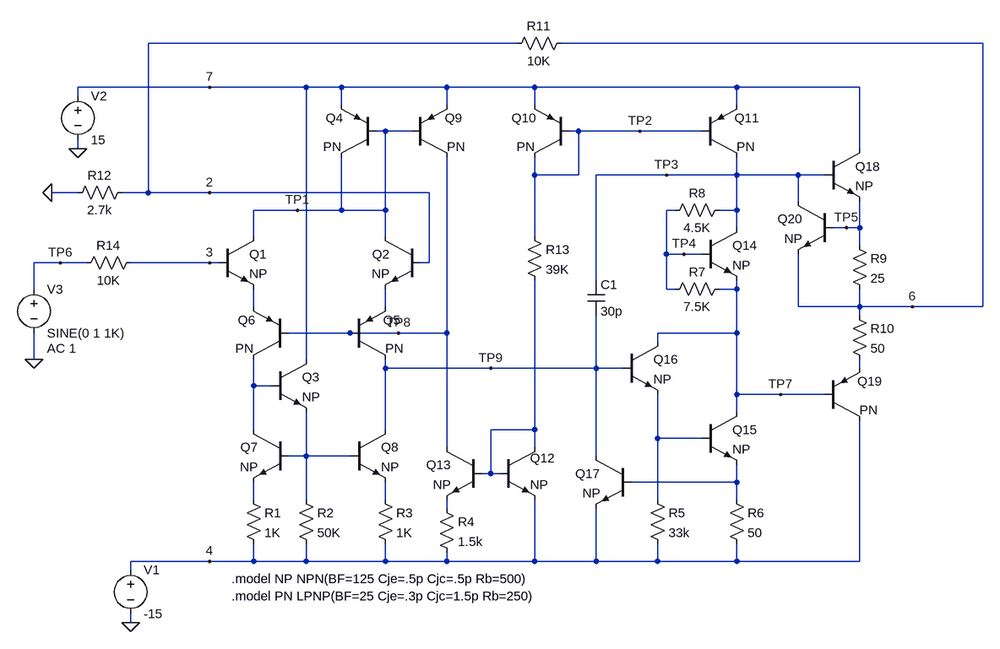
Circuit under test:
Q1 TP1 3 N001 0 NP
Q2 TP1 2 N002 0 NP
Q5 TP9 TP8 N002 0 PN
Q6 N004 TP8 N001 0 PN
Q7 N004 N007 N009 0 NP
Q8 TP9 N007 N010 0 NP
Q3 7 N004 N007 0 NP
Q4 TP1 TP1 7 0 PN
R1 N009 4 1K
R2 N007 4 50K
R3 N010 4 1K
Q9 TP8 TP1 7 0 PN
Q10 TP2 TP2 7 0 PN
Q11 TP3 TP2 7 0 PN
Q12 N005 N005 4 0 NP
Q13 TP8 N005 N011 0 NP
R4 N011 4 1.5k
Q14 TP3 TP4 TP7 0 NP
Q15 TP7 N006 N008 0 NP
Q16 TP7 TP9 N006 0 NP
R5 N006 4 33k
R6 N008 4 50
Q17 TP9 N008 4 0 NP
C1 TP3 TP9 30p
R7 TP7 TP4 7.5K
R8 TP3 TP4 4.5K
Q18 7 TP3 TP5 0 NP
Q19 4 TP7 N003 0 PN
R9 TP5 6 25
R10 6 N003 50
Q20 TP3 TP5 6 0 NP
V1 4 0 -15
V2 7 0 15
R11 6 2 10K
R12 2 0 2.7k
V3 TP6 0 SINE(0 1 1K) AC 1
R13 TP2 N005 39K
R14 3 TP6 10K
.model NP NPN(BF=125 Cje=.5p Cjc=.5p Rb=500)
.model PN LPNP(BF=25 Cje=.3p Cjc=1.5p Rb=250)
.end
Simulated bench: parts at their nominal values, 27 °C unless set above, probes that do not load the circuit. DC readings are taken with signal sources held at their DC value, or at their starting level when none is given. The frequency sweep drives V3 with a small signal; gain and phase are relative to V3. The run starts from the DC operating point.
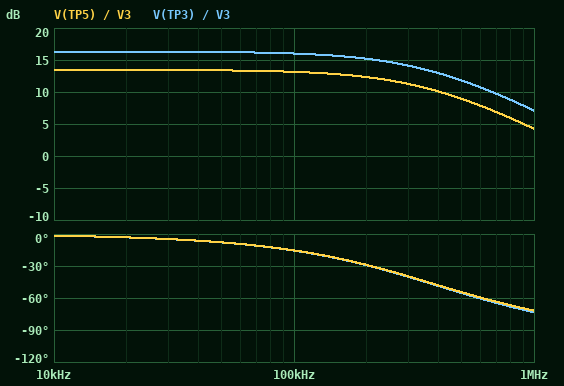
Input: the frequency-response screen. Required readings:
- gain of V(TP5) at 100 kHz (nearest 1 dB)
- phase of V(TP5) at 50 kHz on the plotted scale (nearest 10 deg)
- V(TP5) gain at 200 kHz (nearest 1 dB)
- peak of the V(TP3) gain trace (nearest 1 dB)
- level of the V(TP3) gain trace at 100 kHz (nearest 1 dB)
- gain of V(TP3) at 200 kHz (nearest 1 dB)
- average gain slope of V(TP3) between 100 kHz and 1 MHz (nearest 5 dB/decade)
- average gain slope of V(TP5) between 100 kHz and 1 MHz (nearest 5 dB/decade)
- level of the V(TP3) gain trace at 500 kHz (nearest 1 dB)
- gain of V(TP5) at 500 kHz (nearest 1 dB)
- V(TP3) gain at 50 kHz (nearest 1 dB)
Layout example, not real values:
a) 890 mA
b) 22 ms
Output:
a) 13 dB
b) -10 deg
c) 12 dB
d) 16 dB
e) 16 dB
f) 15 dB
g) -10 dB/decade
h) -10 dB/decade
i) 12 dB
j) 9 dB
k) 16 dB
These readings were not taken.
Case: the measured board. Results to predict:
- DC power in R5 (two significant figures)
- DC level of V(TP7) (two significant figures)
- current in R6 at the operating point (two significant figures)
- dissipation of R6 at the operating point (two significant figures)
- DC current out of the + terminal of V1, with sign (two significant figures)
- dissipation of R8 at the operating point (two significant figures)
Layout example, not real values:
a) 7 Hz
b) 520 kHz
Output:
a) 19 µW
b) -630 mV
c) 650 µA
d) 21 µW
e) -1.5 mA
f) 51 µW
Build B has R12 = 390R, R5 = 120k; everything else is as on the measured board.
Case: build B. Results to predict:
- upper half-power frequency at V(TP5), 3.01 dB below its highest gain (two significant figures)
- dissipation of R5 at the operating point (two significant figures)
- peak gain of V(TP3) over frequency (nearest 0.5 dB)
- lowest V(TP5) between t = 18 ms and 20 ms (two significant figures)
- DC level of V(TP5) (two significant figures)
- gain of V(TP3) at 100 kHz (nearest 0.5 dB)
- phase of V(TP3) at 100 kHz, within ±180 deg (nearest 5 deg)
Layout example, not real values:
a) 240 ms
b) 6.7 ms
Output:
a) 67 kHz
b) 5.3 µW
c) 31.0 dB
d) -13 V
e) -52 mV
f) 26.0 dB
g) -55 deg
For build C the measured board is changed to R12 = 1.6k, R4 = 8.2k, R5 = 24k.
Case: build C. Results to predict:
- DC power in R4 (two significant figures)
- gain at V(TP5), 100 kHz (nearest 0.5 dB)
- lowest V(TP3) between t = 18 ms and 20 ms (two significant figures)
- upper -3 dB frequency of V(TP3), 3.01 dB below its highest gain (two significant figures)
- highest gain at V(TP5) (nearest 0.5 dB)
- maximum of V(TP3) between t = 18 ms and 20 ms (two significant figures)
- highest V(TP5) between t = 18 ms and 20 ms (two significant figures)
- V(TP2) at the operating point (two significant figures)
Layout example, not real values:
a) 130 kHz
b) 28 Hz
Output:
a) 1.4 µW
b) 12.0 dB
c) -6.8 V
d) 64 kHz
e) 17.0 dB
f) 8.0 V
g) 7.3 V
h) 14 V
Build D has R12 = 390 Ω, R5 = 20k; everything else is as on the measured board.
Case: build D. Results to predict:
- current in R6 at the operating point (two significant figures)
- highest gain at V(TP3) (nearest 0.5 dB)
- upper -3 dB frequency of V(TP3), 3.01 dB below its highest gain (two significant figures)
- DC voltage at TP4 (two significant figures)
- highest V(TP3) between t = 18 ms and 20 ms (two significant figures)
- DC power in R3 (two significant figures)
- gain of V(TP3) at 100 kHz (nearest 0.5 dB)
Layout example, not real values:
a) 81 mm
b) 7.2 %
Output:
a) 640 µA
b) 31.5 dB
c) 64 kHz
d) 89 mV
e) 15 V
f) 580 nW
g) 26.0 dB
